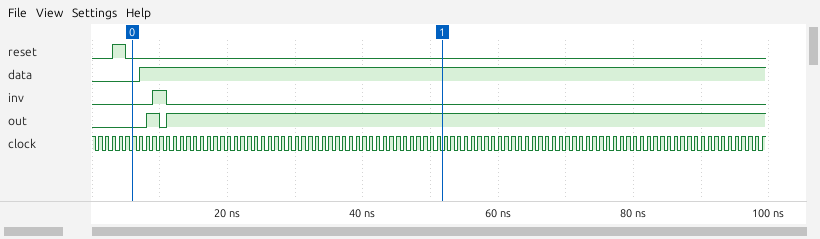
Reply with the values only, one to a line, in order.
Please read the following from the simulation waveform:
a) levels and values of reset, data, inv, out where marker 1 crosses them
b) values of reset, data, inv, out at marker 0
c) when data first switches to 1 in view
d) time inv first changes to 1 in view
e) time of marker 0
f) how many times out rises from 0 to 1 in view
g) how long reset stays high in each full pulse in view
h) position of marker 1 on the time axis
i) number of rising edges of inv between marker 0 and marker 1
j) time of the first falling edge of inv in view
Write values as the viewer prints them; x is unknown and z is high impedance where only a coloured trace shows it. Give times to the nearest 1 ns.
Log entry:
reset=0, data=1, inv=0, out=1
reset=0, data=0, inv=0, out=0
7 ns
9 ns
6 ns
2
2 ns
52 ns
1
11 ns
